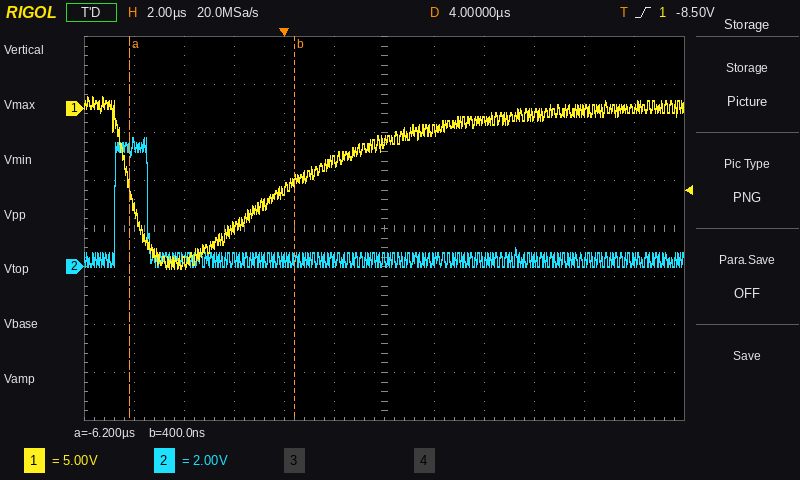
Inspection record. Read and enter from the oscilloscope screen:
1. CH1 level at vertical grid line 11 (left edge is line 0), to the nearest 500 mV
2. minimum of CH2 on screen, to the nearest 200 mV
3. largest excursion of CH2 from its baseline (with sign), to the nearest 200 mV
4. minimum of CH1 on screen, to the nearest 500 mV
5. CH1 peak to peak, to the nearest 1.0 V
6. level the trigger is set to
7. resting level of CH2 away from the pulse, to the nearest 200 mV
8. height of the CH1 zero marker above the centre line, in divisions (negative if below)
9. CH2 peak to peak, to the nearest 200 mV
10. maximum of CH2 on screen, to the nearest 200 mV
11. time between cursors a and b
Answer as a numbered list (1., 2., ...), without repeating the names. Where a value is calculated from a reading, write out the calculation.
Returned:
1. 0.0 V
2. 0.0 V
3. 5.4 V − (400 mV) = +5.0 V
4. -16.5 V
5. 18.0 V
6. -8.50 V
7. 400 mV
8. +2.5 div
9. 5.4 V − (0.0 V) = 5.4 V
10. 5.4 V
11. 400 ns − (-6.2 µs) = 6.6 µs
